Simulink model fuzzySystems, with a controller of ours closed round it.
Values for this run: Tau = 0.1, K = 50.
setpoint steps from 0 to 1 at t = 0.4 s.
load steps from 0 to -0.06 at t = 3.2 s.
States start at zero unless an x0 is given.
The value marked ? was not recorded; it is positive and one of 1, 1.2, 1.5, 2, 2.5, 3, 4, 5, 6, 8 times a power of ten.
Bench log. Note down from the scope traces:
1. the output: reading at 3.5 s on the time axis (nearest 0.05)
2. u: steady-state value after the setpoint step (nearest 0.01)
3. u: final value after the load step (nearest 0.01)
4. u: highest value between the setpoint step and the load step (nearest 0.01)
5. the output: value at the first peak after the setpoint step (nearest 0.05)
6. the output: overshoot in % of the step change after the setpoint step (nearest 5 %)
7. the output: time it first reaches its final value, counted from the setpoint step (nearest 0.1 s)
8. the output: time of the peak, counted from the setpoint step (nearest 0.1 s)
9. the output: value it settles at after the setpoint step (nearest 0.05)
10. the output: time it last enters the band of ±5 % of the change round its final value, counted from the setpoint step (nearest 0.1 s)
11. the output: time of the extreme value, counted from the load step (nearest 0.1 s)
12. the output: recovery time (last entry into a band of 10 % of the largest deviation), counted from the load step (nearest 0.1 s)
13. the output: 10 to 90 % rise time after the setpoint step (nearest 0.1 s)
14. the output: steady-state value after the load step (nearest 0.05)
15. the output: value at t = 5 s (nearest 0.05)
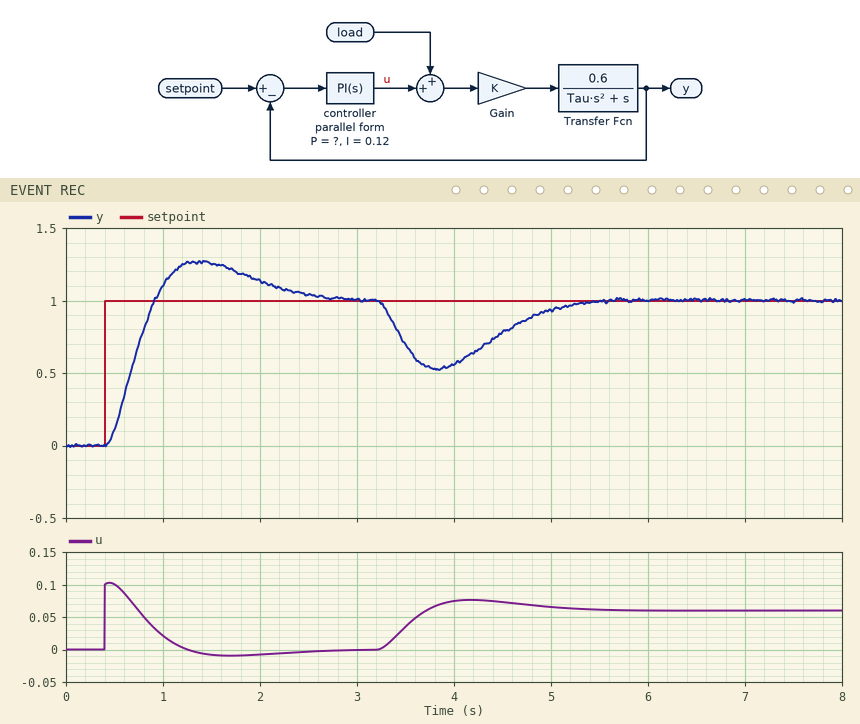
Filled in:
0.70
0.00
0.06
0.10
1.25
25 %
0.5 s
1.0 s
1.00
2.0 s
0.6 s
1.9 s
0.4 s
1.00
0.95
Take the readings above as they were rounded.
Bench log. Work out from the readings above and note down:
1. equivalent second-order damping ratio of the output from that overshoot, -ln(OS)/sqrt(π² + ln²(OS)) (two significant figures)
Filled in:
0.40
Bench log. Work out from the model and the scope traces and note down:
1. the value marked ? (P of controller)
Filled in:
0.1
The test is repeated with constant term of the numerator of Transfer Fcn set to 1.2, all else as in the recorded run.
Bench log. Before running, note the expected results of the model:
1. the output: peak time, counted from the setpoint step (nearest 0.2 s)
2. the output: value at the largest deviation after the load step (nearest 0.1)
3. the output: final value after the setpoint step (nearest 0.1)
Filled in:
0.6 s
0.4
1.0
